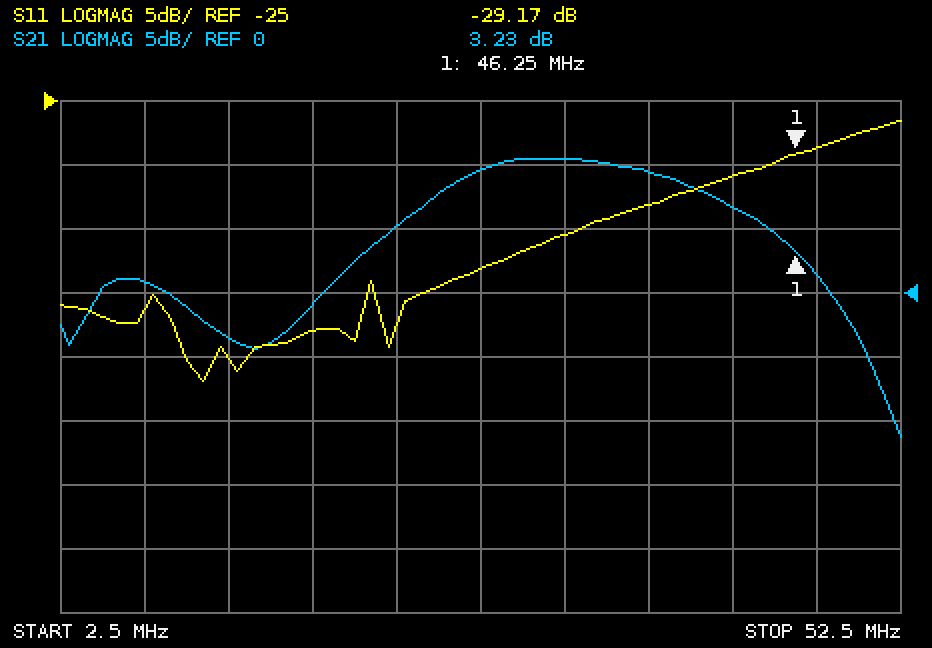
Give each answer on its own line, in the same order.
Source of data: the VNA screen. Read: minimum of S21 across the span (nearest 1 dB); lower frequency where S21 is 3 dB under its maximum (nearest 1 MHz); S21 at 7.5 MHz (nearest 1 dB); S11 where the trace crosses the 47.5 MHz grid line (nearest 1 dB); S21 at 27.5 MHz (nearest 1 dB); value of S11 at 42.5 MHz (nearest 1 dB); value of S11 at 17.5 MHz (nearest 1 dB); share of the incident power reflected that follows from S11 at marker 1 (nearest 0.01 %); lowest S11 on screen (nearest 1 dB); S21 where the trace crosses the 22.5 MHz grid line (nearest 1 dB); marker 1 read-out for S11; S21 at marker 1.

-11 dB
25 MHz
1 dB
-29 dB
10 dB
-31 dB
-43 dB
0.12 %
-47 dB
5 dB
-29.17 dB
3.23 dB
